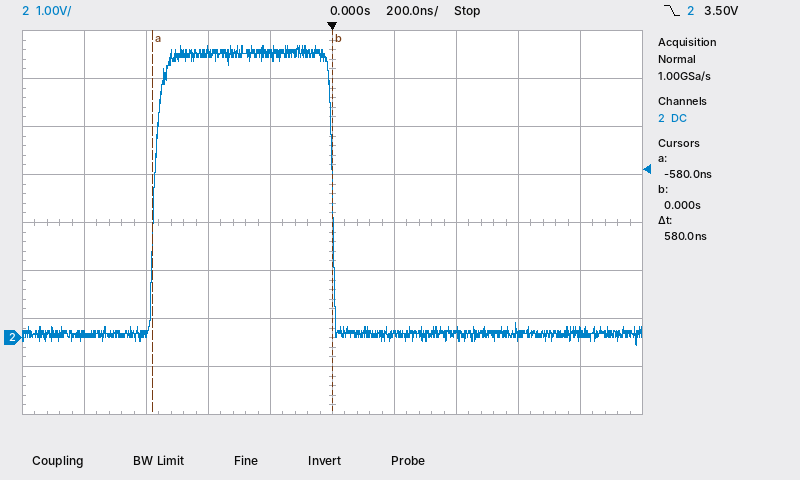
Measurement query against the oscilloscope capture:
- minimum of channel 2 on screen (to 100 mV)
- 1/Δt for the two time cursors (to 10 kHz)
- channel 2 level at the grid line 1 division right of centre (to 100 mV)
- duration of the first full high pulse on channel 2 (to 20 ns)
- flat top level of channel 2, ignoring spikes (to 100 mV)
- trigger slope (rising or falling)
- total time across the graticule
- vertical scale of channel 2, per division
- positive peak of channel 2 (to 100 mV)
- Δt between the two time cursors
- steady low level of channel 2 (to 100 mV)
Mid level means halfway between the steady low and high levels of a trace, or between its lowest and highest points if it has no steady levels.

-200 mV
1.72 MHz
100 mV
580 ns
5.9 V
falling
2 µs
1 V
6.1 V
580 ns
100 mV
